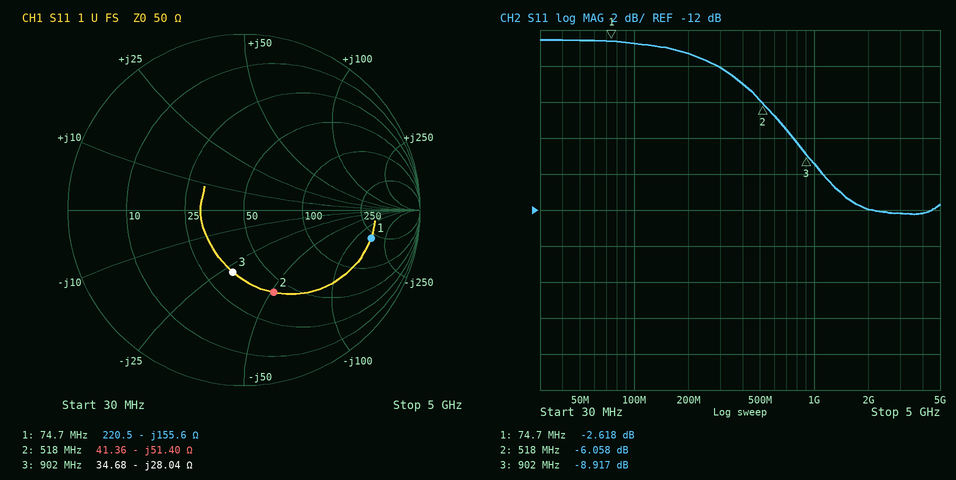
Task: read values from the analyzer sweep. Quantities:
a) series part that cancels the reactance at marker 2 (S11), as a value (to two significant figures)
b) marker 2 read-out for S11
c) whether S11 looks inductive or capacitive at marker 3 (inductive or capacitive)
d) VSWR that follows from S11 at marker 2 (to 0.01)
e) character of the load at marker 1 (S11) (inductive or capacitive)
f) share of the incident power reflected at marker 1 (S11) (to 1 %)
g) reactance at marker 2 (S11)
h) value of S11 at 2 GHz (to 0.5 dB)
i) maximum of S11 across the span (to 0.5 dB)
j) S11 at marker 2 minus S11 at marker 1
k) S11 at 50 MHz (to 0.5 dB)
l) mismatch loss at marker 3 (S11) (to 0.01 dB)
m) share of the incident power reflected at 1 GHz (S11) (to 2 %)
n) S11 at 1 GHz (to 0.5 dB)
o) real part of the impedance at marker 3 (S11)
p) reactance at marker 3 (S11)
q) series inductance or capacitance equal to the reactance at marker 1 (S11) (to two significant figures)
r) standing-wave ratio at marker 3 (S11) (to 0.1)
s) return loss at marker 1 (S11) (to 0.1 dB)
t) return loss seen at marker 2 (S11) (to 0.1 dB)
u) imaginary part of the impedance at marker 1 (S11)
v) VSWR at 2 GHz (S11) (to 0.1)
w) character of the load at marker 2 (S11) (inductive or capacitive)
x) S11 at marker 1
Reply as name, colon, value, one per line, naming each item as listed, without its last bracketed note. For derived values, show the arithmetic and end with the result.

series part that cancels the reactance at marker 2 (S11), as a value: L = 51.4 Ω/(2π × 518 MHz) ≈ 16 nH
marker 2 read-out for S11: -6.058 dB
whether S11 looks inductive or capacitive at marker 3: capacitive
VSWR that follows from S11 at marker 2: (1 + 0.4979)/(1 − 0.4979) ≈ 2.98
character of the load at marker 1 (S11): capacitive
share of the incident power reflected at marker 1 (S11): 10^(-2.618/10) ≈ 55 %
reactance at marker 2: -51.40 Ω
value of S11 at 2 GHz: -12.0 dB
maximum of S11 across the span: -2.5 dB
S11 at marker 2 minus S11 at marker 1: -6.058 − (-2.618) = -3.440 dB
S11 at 50 MHz: -2.5 dB
mismatch loss at marker 3 (S11): −10 log10(1 − 10^(-8.917/10)) ≈ 0.60 dB
share of the incident power reflected at 1 GHz (S11): 10^(-9.5/10) ≈ 11.2 %, so 12 % to the nearest 2 %
S11 at 1 GHz: -9.5 dB
real part of the impedance at marker 3: 34.68 Ω
reactance at marker 3: -28.04 Ω
series inductance or capacitance equal to the reactance at marker 1 (S11): C = 1/(2π × 74.7 MHz × 155.6 Ω) ≈ 14 pF
standing-wave ratio at marker 3 (S11): 2.1
return loss at marker 1 (S11): 2.6 dB
return loss seen at marker 2 (S11): 6.1 dB
imaginary part of the impedance at marker 1: -155.6 Ω
VSWR at 2 GHz (S11): |Γ| = 10^(-12/20) = 0.2512; VSWR = (1 + 0.2512)/(1 − 0.2512) ≈ 1.7
character of the load at marker 2 (S11): capacitive
S11 at marker 1: -2.618 dB
